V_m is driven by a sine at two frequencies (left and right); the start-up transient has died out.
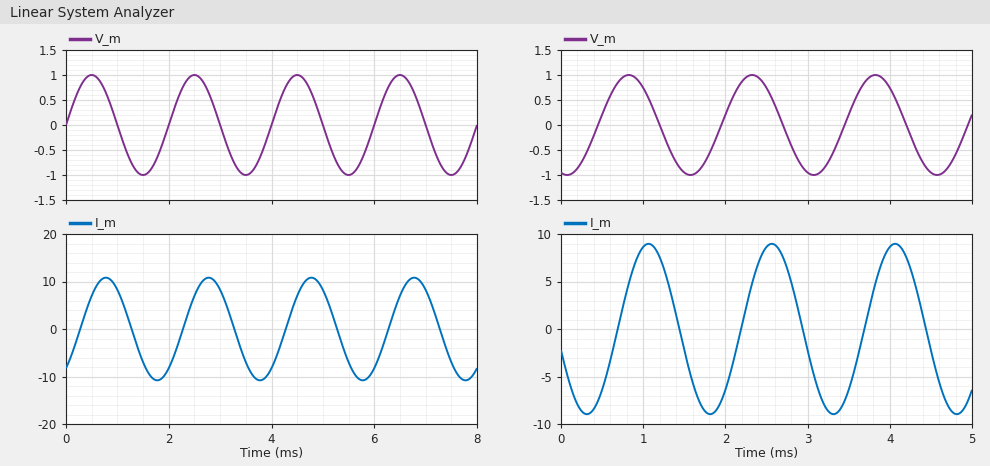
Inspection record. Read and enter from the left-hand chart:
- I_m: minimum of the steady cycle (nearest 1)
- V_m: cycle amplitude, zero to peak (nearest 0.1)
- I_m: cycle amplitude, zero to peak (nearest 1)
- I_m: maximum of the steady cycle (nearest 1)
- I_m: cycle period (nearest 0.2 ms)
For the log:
-11
1.0
11
11
2.0 ms
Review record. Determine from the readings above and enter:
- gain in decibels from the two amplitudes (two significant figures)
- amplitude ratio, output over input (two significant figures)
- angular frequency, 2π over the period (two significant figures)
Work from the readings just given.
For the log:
21 dB
11
3.1 rad/ms
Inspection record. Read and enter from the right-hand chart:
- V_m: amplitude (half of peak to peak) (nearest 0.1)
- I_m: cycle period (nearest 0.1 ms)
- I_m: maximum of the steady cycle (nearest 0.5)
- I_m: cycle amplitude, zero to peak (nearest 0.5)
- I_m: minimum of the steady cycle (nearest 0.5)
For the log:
1.0
1.5 ms
9.0
9.0
-9.0
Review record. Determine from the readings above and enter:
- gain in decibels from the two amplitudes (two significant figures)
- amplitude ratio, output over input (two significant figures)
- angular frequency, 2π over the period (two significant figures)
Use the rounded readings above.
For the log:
19 dB
9.0
4.2 rad/ms
